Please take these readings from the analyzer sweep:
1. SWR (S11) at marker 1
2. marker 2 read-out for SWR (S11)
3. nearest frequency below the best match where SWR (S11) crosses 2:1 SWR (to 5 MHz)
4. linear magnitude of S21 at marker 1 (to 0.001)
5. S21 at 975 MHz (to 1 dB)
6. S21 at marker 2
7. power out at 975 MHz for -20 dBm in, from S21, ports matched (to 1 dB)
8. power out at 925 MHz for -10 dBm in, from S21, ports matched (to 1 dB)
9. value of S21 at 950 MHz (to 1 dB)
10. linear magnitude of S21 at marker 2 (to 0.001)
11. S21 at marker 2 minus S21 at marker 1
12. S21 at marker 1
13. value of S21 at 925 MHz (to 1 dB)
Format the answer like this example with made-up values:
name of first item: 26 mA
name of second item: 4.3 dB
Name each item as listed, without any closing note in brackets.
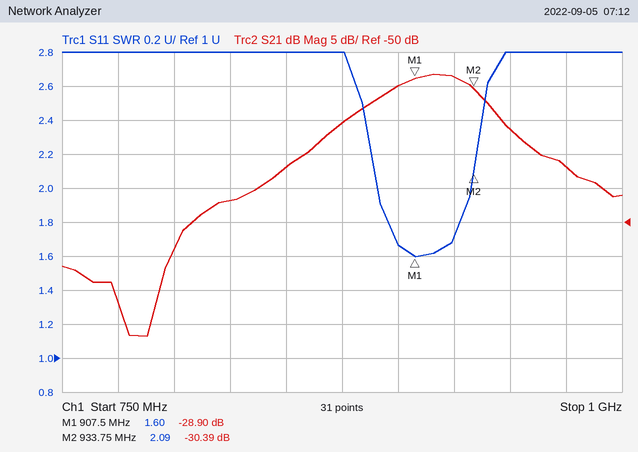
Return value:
SWR (S11) at marker 1: 1.60
marker 2 read-out for SWR: 2.09
nearest frequency below the best match where SWR (S11) crosses 2:1 SWR: 890 MHz
linear magnitude of S21 at marker 1: 0.036
S21 at 975 MHz: -42 dB
S21 at marker 2: -30.39 dB
power out at 975 MHz for -20 dBm in, from S21, ports matched: -62 dBm
power out at 925 MHz for -10 dBm in, from S21, ports matched: -39 dBm
value of S21 at 950 MHz: -36 dB
linear magnitude of S21 at marker 2: 0.030
S21 at marker 2 minus S21 at marker 1: -1.49 dB
S21 at marker 1: -28.90 dB
value of S21 at 925 MHz: -29 dB
